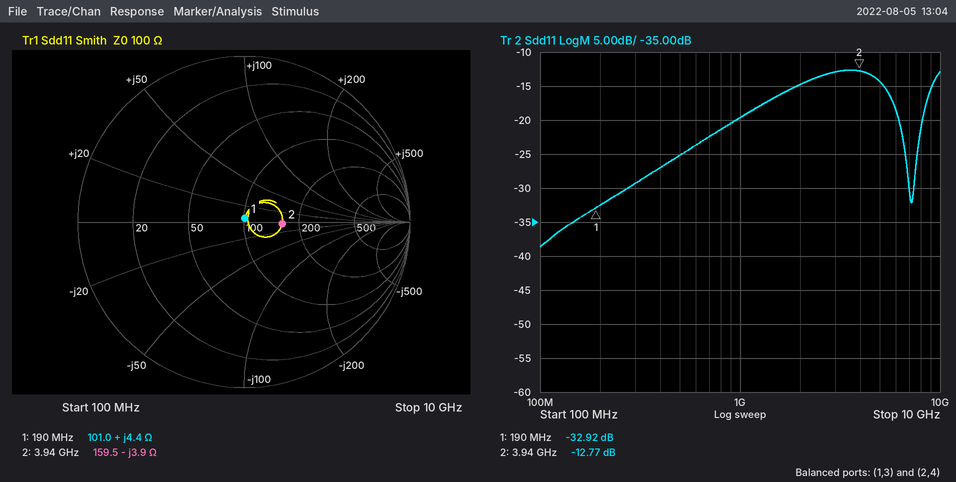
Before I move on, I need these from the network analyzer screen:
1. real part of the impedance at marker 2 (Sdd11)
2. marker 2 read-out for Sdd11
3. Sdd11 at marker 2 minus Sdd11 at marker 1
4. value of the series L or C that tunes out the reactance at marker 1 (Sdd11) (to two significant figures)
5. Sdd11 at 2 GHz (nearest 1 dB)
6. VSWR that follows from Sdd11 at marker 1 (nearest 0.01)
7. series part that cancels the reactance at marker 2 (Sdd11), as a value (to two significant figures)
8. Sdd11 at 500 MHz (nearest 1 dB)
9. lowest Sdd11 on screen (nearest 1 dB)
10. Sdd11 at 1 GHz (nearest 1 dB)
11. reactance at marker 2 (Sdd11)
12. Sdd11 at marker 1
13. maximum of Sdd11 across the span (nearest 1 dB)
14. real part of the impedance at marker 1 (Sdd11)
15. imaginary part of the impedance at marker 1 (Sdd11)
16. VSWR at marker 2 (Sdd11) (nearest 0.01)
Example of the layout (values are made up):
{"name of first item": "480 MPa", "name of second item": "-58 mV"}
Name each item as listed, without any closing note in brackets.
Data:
{"real part of the impedance at marker 2": "159.5 Ω", "marker 2 read-out for Sdd11": "-12.77 dB", "Sdd11 at marker 2 minus Sdd11 at marker 1": "20.15 dB", "value of the series L or C that tunes out the reactance at marker 1 (Sdd11)": "190 pF", "Sdd11 at 2 GHz": "-15 dB", "VSWR that follows from Sdd11 at marker 1": "1.05", "series part that cancels the reactance at marker 2 (Sdd11), as a value": "160 pH", "Sdd11 at 500 MHz": "-25 dB", "lowest Sdd11 on screen": "-39 dB", "Sdd11 at 1 GHz": "-20 dB", "reactance at marker 2": "-3.9 Ω", "Sdd11 at marker 1": "-32.92 dB", "maximum of Sdd11 across the span": "-13 dB", "real part of the impedance at marker 1": "101.0 Ω", "imaginary part of the impedance at marker 1": "+4.4 Ω", "VSWR at marker 2 (Sdd11)": "1.60"}
